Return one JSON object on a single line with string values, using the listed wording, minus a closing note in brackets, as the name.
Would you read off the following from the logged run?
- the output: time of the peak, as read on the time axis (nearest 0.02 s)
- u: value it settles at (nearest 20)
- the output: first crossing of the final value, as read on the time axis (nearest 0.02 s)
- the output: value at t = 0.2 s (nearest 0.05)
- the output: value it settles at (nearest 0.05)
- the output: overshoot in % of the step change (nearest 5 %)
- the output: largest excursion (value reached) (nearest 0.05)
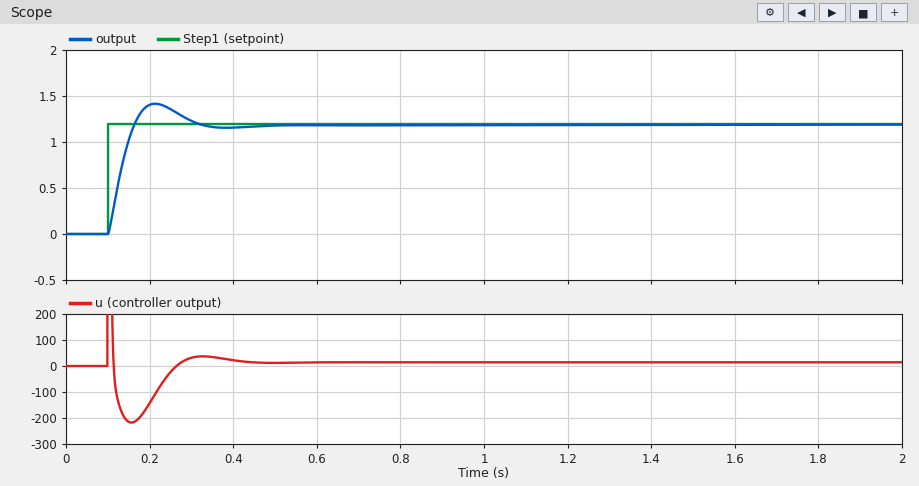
{"the output: time of the peak, as read on the time axis": "0.22 s", "u: value it settles at": "20", "the output: first crossing of the final value, as read on the time axis": "0.16 s", "the output: value at t = 0.2 s": "1.40", "the output: value it settles at": "1.20", "the output: overshoot in % of the step change": "20 %", "the output: largest excursion (value reached)": "1.40"}
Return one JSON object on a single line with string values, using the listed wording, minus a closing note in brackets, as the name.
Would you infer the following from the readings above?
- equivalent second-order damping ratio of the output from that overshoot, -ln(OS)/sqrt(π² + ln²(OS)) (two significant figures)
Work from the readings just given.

{"equivalent second-order damping ratio of the output from that overshoot, -ln(OS)/sqrt(π² + ln²(OS))": "0.46"}
